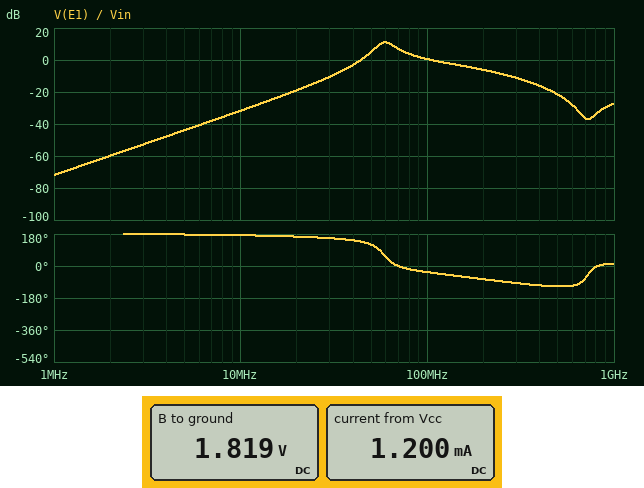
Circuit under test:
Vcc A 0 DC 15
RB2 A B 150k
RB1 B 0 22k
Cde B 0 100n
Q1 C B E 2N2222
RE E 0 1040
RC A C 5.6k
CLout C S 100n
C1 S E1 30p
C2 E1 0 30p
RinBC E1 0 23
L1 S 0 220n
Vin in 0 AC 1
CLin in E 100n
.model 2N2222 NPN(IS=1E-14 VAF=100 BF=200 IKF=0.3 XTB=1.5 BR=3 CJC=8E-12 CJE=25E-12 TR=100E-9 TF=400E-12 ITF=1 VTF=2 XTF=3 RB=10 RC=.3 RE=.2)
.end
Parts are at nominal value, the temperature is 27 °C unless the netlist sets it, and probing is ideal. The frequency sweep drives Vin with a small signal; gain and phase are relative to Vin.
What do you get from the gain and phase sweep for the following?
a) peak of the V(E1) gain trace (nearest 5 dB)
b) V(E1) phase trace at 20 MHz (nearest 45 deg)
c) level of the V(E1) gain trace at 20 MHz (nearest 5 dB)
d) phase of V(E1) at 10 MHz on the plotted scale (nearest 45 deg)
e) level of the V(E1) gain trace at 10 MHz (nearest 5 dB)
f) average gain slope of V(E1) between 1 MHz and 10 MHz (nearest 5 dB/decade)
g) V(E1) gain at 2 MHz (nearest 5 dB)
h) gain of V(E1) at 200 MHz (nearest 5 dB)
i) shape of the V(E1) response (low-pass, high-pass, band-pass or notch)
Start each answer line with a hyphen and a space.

- 10 dB
- 180 deg
- -20 dB
- 180 deg
- -30 dB
- 40 dB/decade
- -60 dB
- -5 dB
- band-pass
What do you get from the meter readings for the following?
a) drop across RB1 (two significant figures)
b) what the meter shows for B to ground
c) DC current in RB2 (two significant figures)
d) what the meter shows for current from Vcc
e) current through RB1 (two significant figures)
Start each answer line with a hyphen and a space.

- 1.8 V
- 1.819 V
- 88 µA
- 1.200 mA
- 83 µA
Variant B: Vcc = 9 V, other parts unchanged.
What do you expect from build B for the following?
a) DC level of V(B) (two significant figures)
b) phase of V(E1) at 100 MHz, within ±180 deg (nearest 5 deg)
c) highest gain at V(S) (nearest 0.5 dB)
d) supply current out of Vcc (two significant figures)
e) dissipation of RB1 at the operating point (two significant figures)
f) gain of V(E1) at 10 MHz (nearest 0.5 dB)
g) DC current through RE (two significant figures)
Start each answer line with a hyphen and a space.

- 1.1 V
- -30 deg
- 16.5 dB
- 510 µA
- 56 µW
- -39.5 dB
- 460 µA
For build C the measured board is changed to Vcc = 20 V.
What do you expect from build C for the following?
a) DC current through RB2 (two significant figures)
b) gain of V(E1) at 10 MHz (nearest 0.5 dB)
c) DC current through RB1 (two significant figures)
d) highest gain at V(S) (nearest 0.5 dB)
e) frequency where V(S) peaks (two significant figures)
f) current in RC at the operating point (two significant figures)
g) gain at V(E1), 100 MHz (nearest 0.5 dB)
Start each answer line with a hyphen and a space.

- 120 µA
- -28.0 dB
- 110 µA
- 27.0 dB
- 58 MHz
- 1.7 mA
- 3.5 dB
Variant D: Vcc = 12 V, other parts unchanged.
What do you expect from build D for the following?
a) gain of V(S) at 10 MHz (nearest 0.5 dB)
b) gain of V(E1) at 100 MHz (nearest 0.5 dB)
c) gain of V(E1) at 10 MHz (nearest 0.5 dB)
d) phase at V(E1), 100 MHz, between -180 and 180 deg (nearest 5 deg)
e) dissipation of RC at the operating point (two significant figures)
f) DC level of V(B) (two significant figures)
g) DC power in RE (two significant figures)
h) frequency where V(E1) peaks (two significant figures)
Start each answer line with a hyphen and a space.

- -7.5 dB
- -2.5 dB
- -34.5 dB
- -35 deg
- 3.4 mW
- 1.5 V
- 640 µW
- 60 MHz
